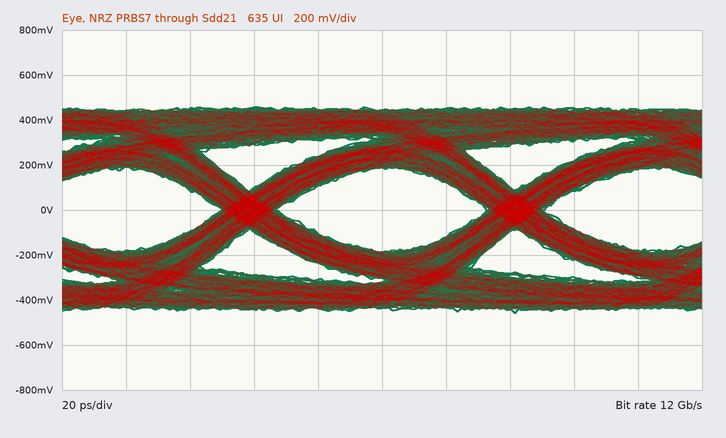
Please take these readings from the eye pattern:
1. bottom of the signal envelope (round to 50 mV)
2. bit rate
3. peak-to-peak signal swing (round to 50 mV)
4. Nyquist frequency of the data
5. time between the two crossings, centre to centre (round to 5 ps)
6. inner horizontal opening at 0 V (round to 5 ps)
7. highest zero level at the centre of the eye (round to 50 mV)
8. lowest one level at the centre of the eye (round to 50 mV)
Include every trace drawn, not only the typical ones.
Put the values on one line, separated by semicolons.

-450 mV; 12 Gb/s; 900 mV; 6 GHz; 85 ps; 65 ps; -200 mV; 200 mV
